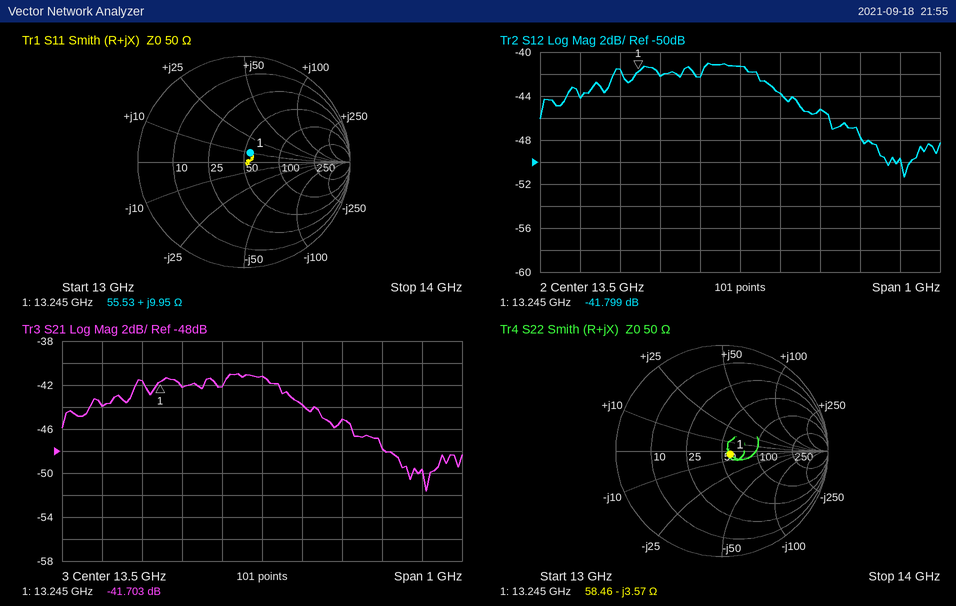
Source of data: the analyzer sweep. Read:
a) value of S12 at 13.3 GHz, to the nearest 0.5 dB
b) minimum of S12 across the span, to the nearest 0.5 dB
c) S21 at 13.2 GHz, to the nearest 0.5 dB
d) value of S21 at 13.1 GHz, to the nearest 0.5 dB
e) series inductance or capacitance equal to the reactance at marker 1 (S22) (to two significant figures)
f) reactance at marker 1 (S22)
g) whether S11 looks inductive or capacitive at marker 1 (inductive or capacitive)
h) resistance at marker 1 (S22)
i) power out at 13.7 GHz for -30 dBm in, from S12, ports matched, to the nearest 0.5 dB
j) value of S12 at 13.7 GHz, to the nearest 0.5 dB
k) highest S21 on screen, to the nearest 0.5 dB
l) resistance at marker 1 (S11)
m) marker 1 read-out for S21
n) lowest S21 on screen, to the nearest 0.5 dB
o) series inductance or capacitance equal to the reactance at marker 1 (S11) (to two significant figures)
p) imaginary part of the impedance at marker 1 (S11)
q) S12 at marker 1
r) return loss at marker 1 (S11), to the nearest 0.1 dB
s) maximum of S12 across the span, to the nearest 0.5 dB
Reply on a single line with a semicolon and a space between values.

-42.0 dB; -51.5 dB; -41.5 dB; -44.0 dB; 3.4 pF; -3.57 Ω; inductive; 58.46 Ω; -75.0 dBm; -45.0 dB; -41.0 dB; 55.53 Ω; -41.703 dB; -51.5 dB; 120 pH; +9.95 Ω; -41.799 dB; 19.4 dB; -41.0 dB
